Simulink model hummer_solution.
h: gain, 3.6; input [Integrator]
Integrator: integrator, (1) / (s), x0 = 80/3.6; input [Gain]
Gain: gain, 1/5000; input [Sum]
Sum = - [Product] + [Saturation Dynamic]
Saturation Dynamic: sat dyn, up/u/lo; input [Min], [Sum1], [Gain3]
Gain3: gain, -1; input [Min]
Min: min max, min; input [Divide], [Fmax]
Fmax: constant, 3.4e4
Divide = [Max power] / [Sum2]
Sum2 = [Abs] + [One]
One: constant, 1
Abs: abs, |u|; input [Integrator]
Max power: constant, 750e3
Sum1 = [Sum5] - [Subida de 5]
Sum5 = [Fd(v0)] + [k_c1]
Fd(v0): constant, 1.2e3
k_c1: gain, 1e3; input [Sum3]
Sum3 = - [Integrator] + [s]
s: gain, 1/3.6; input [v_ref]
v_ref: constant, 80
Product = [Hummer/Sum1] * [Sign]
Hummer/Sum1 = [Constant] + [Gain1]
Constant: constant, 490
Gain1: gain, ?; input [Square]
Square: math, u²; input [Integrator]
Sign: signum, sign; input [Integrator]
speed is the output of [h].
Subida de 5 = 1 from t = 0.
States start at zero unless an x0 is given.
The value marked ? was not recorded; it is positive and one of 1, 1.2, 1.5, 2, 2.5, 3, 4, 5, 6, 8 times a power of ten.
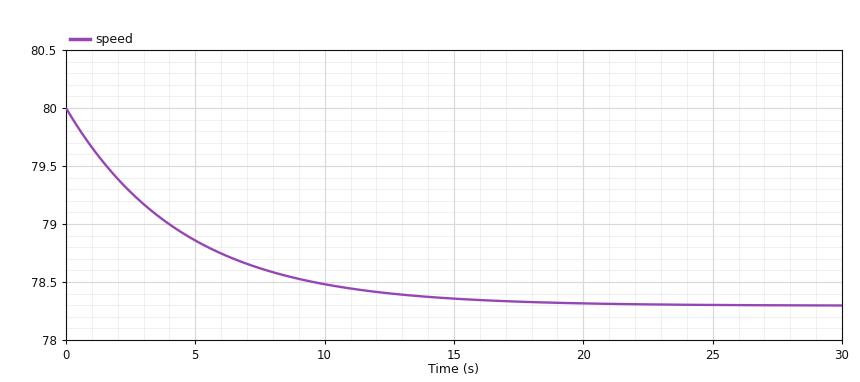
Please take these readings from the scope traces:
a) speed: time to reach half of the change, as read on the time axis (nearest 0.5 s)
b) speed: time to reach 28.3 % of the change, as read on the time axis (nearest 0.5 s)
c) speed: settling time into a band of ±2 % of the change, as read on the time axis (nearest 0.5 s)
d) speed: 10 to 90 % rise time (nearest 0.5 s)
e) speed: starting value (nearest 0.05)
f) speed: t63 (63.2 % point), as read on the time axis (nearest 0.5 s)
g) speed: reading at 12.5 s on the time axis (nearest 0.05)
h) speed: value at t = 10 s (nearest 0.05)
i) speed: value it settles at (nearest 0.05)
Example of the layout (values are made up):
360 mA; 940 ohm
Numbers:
3.0 s; 1.5 s; 17.5 s; 10.0 s; 80.00; 4.5 s; 78.40; 78.50; 78.30
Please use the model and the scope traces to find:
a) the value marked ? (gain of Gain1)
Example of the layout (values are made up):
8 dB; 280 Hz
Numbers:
2.5
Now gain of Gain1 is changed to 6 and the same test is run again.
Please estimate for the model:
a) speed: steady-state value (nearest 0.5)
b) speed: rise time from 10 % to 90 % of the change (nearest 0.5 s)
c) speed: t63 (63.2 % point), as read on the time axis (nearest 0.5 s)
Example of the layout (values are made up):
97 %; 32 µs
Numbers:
73.5; 9.0 s; 4.0 s
